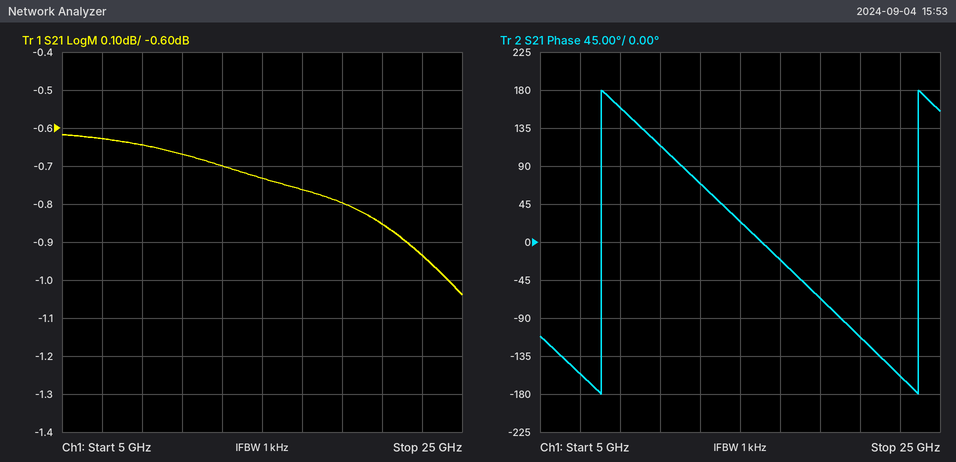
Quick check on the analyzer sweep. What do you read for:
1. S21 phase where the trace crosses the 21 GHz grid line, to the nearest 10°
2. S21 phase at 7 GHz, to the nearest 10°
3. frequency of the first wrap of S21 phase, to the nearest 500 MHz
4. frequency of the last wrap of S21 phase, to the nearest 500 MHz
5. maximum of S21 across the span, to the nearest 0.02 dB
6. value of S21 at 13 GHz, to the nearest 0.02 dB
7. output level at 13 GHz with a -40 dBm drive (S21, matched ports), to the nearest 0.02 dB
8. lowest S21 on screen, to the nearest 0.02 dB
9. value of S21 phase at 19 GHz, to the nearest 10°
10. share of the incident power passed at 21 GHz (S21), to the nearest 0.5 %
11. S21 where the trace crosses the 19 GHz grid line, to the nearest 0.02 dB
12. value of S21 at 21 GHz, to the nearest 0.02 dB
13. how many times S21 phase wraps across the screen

-110°
-160°
8.0 GHz
24.0 GHz
-0.62 dB
-0.70 dB
-40.70 dBm
-1.04 dB
-70°
82.0 %
-0.80 dB
-0.86 dB
2
